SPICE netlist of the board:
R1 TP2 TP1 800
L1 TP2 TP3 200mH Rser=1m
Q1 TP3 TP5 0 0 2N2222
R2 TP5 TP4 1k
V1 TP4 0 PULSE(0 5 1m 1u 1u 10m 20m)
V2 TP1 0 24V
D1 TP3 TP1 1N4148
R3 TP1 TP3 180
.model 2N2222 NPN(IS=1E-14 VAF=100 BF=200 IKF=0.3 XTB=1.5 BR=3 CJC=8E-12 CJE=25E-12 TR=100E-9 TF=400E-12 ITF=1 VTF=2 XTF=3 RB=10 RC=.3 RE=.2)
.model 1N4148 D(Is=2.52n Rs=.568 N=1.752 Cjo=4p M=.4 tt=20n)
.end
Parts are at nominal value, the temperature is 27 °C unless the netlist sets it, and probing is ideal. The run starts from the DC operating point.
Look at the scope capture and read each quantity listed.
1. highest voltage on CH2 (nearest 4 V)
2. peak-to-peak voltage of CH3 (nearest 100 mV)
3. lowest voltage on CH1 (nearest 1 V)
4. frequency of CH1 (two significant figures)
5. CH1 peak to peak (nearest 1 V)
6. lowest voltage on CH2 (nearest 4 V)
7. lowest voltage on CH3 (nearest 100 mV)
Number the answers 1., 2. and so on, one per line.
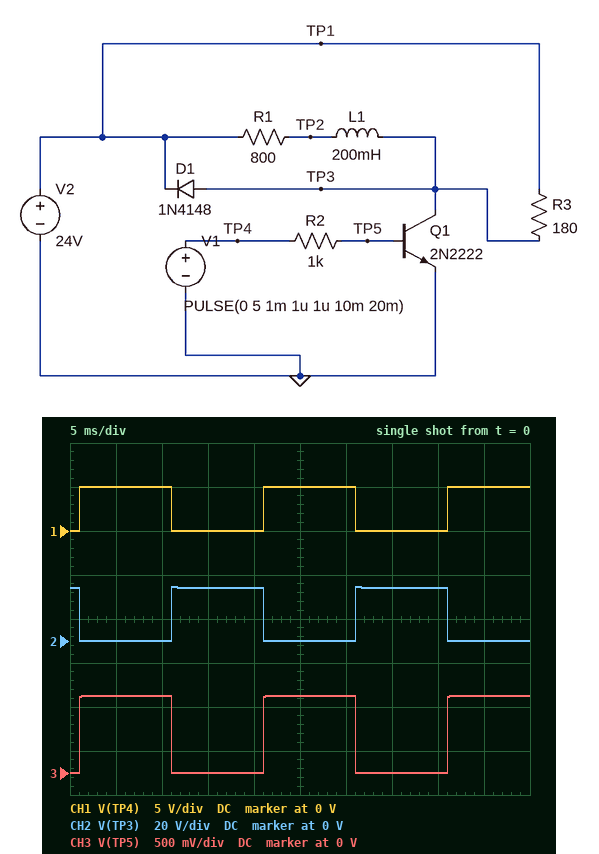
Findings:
1. 24 V
2. 900 mV
3. 0 V
4. 50 Hz
5. 5 V
6. 0 V
7. 0 V
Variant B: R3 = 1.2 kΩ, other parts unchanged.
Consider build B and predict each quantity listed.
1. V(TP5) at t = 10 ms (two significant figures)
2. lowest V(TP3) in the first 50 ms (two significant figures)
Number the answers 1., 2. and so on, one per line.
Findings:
1. 820 mV
2. 42 mV
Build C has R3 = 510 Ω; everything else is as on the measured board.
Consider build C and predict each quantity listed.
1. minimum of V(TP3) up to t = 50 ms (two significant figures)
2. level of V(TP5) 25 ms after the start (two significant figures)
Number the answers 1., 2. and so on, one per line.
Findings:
1. 72 mV
2. 840 mV
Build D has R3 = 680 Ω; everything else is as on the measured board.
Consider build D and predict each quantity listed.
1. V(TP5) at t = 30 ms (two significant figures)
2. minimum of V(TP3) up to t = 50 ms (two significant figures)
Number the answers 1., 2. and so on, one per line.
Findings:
1. 830 mV
2. 60 mV
